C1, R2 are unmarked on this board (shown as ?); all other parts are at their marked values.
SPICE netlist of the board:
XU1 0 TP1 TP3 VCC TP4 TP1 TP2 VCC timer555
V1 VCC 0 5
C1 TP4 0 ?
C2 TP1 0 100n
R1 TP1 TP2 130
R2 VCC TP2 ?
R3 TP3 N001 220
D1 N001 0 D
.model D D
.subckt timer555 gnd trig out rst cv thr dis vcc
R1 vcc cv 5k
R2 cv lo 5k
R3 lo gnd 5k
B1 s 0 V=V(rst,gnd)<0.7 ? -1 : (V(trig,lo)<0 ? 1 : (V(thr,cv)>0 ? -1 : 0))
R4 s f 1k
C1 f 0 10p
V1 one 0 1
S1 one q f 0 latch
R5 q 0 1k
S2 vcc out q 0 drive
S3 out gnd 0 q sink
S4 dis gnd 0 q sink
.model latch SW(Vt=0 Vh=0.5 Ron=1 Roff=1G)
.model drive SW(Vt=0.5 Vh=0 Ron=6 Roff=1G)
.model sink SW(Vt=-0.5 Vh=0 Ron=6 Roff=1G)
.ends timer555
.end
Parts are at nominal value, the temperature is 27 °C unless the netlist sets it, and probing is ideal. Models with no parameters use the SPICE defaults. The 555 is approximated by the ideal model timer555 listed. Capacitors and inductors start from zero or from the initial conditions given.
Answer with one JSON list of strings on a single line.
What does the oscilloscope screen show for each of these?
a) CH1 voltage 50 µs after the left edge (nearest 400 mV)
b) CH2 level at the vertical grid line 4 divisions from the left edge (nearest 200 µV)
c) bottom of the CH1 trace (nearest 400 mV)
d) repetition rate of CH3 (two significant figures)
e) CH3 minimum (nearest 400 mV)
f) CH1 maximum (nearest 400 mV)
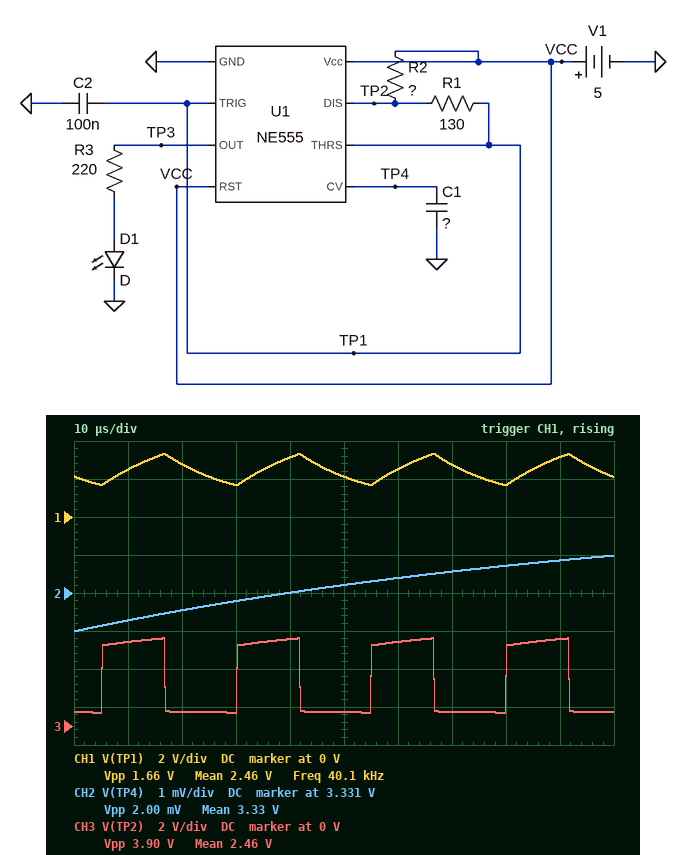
["2.0 V", "3.3310 V", "1.6 V", "40 kHz", "800 mV", "3.2 V"]
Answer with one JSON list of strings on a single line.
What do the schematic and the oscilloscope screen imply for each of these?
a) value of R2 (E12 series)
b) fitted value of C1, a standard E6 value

["39 Ω", "33 nF"]
